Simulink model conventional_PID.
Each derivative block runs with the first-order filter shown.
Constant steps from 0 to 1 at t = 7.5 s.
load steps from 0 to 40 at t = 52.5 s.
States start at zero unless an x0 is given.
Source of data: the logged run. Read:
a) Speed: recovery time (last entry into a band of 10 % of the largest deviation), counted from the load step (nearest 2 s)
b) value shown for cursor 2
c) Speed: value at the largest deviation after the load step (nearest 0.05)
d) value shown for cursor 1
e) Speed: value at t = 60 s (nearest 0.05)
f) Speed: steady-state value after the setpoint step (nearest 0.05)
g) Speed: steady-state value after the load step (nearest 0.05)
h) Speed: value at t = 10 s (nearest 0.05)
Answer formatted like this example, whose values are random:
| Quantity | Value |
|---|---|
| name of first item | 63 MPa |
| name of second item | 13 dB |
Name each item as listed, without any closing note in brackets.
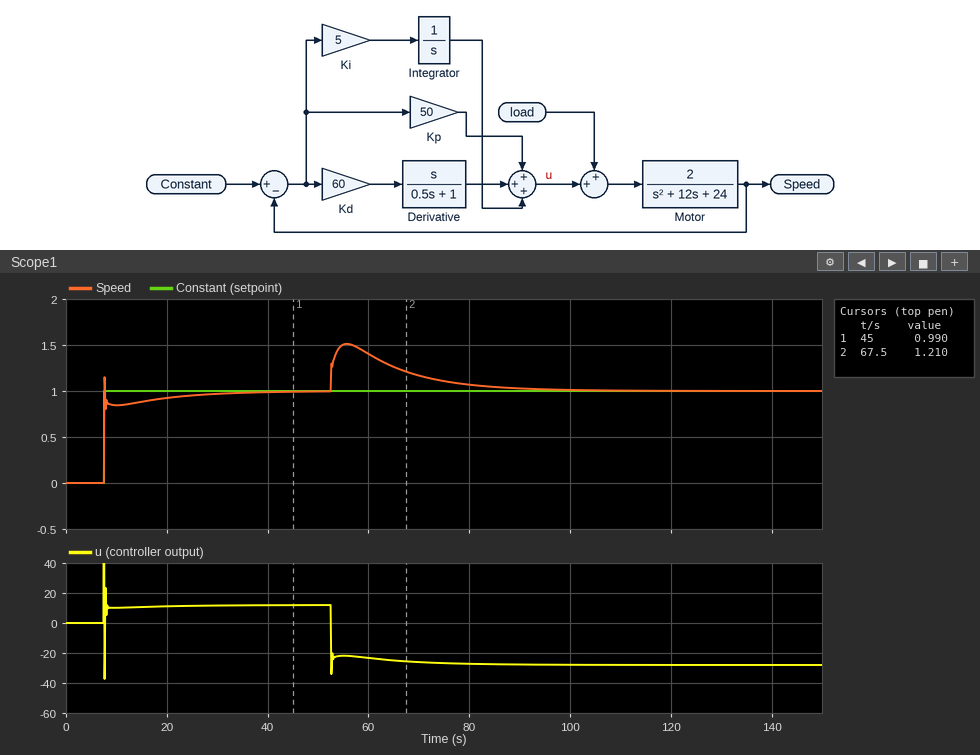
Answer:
| Quantity | Value |
|---|---|
| Speed: recovery time (last entry into a band of 10 % of the largest deviation), counted from the load step | 30 s |
| value shown for cursor 2 | 1.210 |
| Speed: value at the largest deviation after the load step | 1.50 |
| value shown for cursor 1 | 0.990 |
| Speed: value at t = 60 s | 1.40 |
| Speed: steady-state value after the setpoint step | 1.00 |
| Speed: steady-state value after the load step | 1.00 |
| Speed: value at t = 10 s | 0.85 |
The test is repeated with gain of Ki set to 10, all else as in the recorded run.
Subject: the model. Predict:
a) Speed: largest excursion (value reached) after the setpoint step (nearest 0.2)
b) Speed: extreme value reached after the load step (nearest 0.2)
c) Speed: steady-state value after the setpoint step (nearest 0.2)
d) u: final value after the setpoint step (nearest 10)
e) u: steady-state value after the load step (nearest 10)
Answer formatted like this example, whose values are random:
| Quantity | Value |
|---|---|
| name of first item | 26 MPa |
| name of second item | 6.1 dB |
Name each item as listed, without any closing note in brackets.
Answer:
| Quantity | Value |
|---|---|
| Speed: largest excursion (value reached) after the setpoint step | 1.2 |
| Speed: extreme value reached after the load step | 1.4 |
| Speed: steady-state value after the setpoint step | 1.0 |
| u: final value after the setpoint step | 10 |
| u: steady-state value after the load step | -30 |
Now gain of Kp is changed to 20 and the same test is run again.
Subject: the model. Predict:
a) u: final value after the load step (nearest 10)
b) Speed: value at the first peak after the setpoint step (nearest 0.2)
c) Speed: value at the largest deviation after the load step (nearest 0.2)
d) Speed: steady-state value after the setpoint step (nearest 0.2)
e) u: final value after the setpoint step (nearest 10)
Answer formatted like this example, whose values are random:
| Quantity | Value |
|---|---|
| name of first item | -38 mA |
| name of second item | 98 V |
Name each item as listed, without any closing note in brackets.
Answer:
| Quantity | Value |
|---|---|
| u: final value after the load step | -30 |
| Speed: value at the first peak after the setpoint step | 1.0 |
| Speed: value at the largest deviation after the load step | 1.8 |
| Speed: steady-state value after the setpoint step | 1.0 |
| u: final value after the setpoint step | 10 |
